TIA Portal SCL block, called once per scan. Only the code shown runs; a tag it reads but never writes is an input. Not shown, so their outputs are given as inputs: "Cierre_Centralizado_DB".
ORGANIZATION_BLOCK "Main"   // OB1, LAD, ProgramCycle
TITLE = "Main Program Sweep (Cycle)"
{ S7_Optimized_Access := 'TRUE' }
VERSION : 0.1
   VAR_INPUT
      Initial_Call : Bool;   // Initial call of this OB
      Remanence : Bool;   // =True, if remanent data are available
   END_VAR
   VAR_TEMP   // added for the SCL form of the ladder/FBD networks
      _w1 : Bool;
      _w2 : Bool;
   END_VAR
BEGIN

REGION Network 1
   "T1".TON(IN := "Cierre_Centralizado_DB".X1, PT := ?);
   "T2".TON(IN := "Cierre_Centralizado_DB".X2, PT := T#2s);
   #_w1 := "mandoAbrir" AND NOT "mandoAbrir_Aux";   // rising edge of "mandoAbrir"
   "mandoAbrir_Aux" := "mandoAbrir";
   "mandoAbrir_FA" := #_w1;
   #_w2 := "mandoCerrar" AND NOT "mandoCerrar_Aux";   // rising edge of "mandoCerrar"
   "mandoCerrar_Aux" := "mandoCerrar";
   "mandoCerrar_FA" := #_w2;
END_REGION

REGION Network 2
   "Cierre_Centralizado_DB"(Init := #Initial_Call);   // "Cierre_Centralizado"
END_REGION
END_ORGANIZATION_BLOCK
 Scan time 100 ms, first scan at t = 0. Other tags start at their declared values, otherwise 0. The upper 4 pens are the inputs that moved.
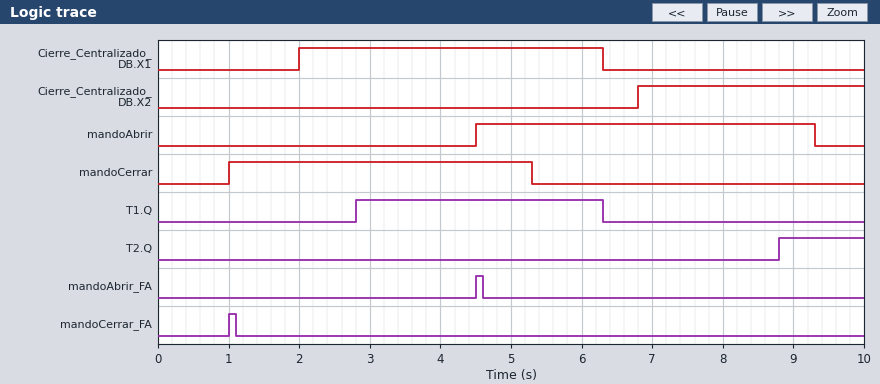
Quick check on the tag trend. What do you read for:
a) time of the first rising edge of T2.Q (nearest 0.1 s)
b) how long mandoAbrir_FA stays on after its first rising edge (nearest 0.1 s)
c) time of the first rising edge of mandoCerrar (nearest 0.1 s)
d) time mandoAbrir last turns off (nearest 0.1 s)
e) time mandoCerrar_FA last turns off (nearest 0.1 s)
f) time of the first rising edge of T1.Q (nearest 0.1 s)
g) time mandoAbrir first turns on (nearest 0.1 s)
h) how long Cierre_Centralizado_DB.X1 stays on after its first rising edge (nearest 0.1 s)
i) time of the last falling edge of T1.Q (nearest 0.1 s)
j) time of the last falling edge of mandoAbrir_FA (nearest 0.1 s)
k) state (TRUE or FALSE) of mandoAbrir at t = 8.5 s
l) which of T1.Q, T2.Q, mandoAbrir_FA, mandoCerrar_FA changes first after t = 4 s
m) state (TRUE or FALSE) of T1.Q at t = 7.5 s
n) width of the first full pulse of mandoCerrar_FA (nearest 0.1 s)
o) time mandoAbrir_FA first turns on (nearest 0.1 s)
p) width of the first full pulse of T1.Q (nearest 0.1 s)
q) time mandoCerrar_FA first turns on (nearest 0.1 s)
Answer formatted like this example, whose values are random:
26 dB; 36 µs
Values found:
8.8 s; 0.1 s; 1.0 s; 9.3 s; 1.1 s; 2.8 s; 4.5 s; 4.3 s; 6.3 s; 4.6 s; TRUE; mandoAbrir_FA; FALSE; 0.1 s; 4.5 s; 3.5 s; 1.0 s
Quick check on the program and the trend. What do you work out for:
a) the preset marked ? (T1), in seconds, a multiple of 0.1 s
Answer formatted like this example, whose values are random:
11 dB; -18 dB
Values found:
0.8 s
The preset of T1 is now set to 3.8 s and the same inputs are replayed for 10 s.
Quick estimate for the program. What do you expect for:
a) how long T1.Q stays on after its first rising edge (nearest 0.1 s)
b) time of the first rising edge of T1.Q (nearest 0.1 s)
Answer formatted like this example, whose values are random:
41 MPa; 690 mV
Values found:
0.5 s; 5.8 s
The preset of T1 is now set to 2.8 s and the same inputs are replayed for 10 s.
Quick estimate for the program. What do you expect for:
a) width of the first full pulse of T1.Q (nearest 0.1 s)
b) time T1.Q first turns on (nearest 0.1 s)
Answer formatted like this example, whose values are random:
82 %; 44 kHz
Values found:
1.5 s; 4.8 s
